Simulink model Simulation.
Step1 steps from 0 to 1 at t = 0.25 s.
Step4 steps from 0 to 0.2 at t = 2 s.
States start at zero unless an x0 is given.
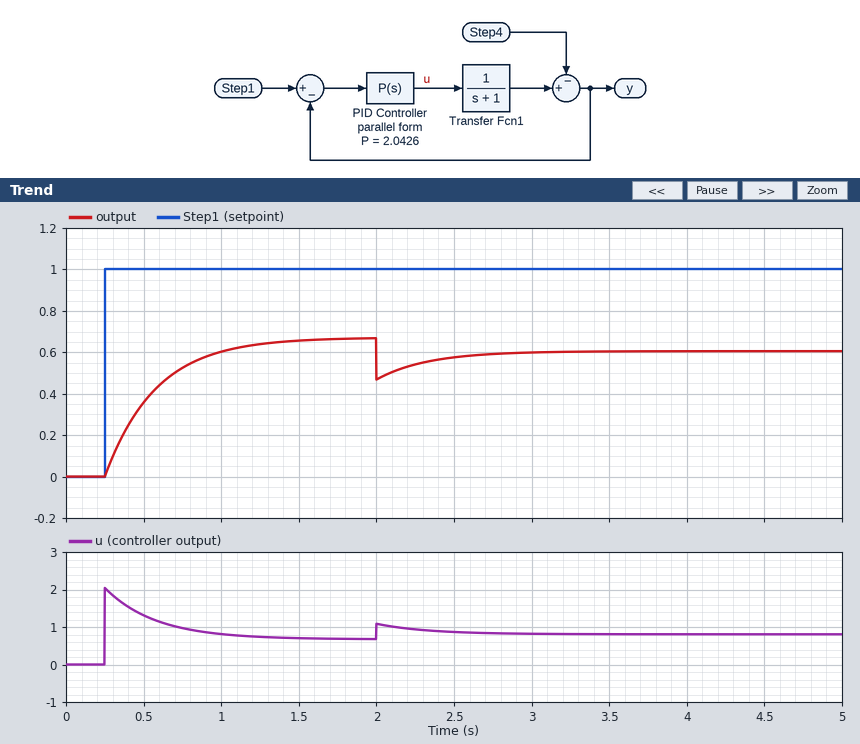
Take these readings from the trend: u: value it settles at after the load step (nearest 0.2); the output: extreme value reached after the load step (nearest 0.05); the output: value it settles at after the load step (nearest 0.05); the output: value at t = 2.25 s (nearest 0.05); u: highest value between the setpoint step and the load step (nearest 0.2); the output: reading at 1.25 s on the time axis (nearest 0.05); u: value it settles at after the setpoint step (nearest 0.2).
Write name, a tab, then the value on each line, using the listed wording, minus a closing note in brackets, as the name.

u: value it settles at after the load step	0.8
the output: extreme value reached after the load step	0.45
the output: value it settles at after the load step	0.60
the output: value at t = 2.25 s	0.55
u: highest value between the setpoint step and the load step	2.0
the output: reading at 1.25 s on the time axis	0.65
u: value it settles at after the setpoint step	0.6
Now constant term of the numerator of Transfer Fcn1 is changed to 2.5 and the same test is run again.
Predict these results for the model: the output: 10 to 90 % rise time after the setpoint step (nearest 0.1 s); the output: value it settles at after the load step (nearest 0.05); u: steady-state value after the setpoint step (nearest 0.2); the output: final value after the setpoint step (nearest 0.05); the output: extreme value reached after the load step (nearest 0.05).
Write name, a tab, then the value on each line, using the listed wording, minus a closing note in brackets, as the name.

the output: 10 to 90 % rise time after the setpoint step	0.4 s
the output: value it settles at after the load step	0.80
u: steady-state value after the setpoint step	0.4
the output: final value after the setpoint step	0.85
the output: extreme value reached after the load step	0.65
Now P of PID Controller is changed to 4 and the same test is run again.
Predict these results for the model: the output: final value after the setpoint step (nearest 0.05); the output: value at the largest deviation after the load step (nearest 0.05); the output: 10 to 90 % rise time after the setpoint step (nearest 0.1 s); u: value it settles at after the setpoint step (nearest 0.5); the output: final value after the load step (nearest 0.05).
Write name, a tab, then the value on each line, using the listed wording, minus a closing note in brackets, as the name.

the output: final value after the setpoint step	0.80
the output: value at the largest deviation after the load step	0.60
the output: 10 to 90 % rise time after the setpoint step	0.4 s
u: value it settles at after the setpoint step	1.0
the output: final value after the load step	0.75
